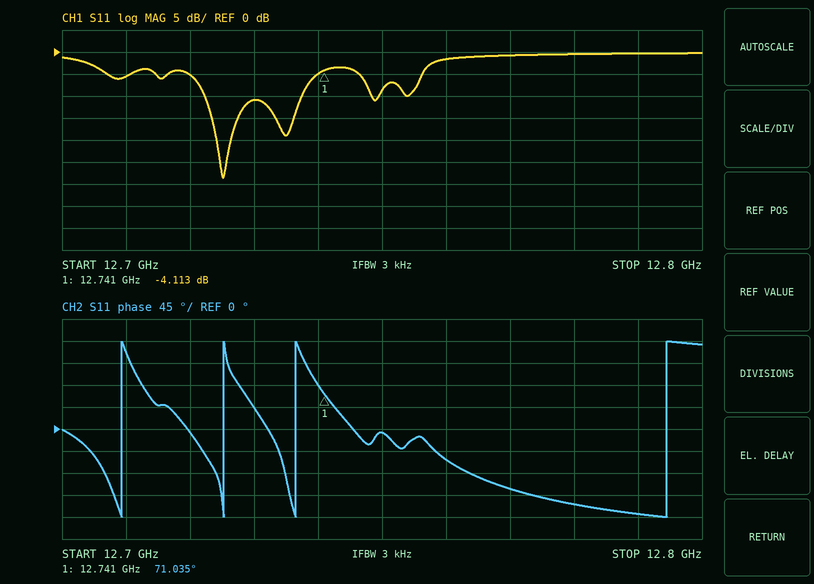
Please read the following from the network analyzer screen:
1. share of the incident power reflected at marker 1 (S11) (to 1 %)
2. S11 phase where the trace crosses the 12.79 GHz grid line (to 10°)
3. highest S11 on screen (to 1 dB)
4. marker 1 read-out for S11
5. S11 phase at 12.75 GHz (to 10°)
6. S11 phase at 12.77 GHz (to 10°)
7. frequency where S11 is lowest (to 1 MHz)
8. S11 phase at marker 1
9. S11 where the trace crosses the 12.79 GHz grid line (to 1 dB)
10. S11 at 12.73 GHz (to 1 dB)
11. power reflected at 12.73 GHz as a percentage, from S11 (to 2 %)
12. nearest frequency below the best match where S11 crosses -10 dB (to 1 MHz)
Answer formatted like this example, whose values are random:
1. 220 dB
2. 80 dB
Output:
1. 39 %
2. -170°
3. 0 dB
4. -4.113 dB
5. -10°
6. -120°
7. 12.725 GHz
8. 71.035°
9. 0 dB
10. -11 dB
11. 8 %
12. 12.722 GHz
